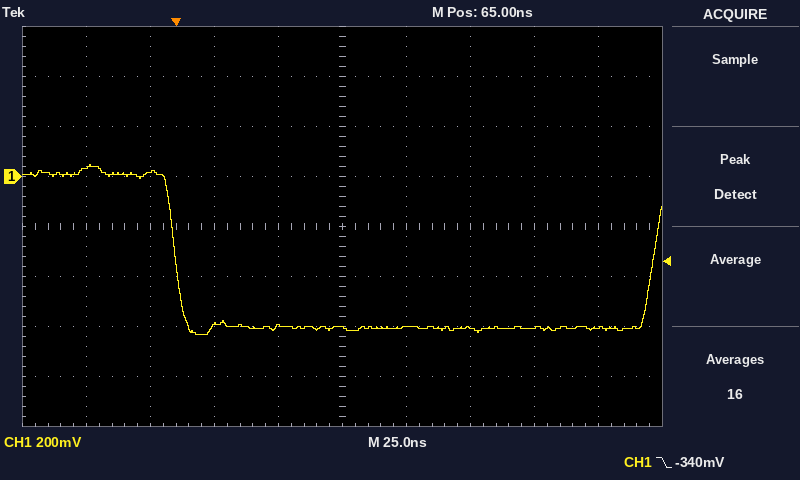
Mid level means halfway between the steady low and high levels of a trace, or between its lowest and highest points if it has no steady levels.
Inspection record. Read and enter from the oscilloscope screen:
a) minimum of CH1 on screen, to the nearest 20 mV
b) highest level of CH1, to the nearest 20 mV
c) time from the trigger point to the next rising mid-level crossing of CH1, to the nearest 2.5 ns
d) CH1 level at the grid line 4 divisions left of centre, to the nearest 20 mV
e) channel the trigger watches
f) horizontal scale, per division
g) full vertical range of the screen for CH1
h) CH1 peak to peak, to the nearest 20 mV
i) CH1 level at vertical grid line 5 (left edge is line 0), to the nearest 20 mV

-640 mV
40 mV
187.5 ns
40 mV
CH1
25 ns
1.6 V
680 mV
-600 mV
